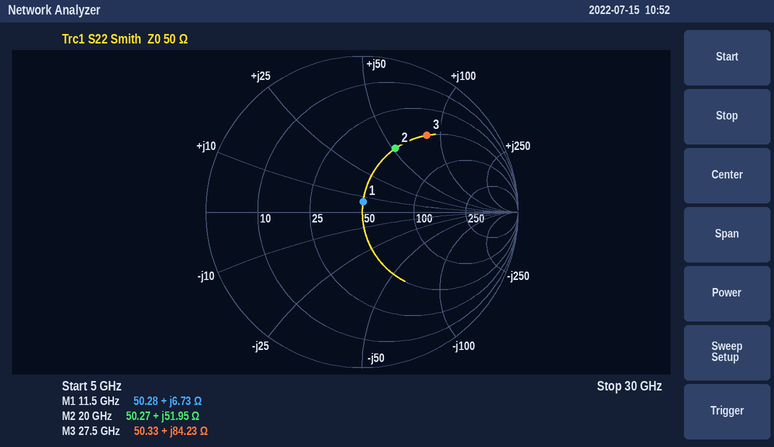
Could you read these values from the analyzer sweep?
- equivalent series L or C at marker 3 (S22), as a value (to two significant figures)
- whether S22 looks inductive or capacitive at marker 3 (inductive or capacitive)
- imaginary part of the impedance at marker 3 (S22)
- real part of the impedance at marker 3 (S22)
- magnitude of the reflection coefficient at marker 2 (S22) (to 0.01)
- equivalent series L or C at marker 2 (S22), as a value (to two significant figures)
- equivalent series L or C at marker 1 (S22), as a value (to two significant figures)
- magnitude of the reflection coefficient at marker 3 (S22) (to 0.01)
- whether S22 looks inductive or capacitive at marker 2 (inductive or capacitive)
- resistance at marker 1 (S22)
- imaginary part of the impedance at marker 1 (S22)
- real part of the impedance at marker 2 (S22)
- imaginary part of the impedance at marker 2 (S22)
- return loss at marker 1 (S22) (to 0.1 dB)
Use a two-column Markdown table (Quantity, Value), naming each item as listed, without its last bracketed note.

| Quantity | Value |
|---|---|
| equivalent series L or C at marker 3 (S22), as a value | 490 pH |
| whether S22 looks inductive or capacitive at marker 3 | inductive |
| imaginary part of the impedance at marker 3 | +84.23 Ω |
| real part of the impedance at marker 3 | 50.33 Ω |
| magnitude of the reflection coefficient at marker 2 (S22) | 0.46 |
| equivalent series L or C at marker 2 (S22), as a value | 410 pH |
| equivalent series L or C at marker 1 (S22), as a value | 93 pH |
| magnitude of the reflection coefficient at marker 3 (S22) | 0.64 |
| whether S22 looks inductive or capacitive at marker 2 | inductive |
| resistance at marker 1 | 50.28 Ω |
| imaginary part of the impedance at marker 1 | +6.73 Ω |
| real part of the impedance at marker 2 | 50.27 Ω |
| imaginary part of the impedance at marker 2 | +51.95 Ω |
| return loss at marker 1 (S22) | 23.5 dB |
